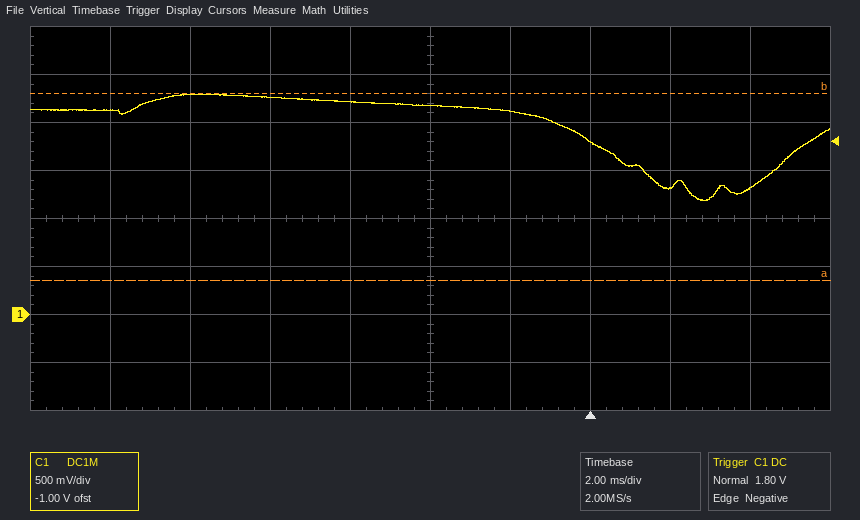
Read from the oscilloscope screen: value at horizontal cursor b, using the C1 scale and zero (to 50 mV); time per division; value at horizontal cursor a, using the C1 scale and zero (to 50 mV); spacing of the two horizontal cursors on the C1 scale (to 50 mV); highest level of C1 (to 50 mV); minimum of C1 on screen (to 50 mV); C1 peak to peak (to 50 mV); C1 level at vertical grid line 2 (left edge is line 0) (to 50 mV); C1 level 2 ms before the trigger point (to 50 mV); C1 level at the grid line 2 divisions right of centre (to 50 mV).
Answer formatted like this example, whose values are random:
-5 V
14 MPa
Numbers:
2.30 V
2 ms
350 mV
1.95 V
2.30 V
1.20 V
1.10 V
2.30 V
2.10 V
1.80 V
